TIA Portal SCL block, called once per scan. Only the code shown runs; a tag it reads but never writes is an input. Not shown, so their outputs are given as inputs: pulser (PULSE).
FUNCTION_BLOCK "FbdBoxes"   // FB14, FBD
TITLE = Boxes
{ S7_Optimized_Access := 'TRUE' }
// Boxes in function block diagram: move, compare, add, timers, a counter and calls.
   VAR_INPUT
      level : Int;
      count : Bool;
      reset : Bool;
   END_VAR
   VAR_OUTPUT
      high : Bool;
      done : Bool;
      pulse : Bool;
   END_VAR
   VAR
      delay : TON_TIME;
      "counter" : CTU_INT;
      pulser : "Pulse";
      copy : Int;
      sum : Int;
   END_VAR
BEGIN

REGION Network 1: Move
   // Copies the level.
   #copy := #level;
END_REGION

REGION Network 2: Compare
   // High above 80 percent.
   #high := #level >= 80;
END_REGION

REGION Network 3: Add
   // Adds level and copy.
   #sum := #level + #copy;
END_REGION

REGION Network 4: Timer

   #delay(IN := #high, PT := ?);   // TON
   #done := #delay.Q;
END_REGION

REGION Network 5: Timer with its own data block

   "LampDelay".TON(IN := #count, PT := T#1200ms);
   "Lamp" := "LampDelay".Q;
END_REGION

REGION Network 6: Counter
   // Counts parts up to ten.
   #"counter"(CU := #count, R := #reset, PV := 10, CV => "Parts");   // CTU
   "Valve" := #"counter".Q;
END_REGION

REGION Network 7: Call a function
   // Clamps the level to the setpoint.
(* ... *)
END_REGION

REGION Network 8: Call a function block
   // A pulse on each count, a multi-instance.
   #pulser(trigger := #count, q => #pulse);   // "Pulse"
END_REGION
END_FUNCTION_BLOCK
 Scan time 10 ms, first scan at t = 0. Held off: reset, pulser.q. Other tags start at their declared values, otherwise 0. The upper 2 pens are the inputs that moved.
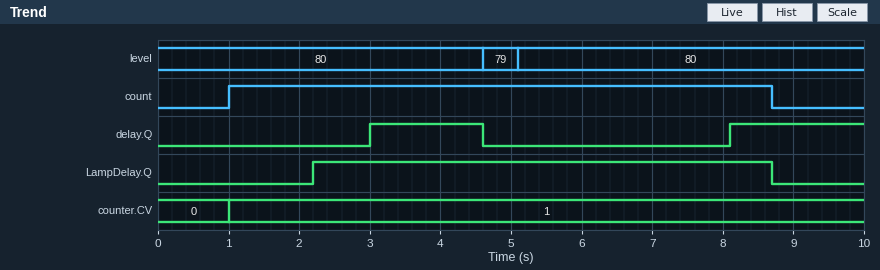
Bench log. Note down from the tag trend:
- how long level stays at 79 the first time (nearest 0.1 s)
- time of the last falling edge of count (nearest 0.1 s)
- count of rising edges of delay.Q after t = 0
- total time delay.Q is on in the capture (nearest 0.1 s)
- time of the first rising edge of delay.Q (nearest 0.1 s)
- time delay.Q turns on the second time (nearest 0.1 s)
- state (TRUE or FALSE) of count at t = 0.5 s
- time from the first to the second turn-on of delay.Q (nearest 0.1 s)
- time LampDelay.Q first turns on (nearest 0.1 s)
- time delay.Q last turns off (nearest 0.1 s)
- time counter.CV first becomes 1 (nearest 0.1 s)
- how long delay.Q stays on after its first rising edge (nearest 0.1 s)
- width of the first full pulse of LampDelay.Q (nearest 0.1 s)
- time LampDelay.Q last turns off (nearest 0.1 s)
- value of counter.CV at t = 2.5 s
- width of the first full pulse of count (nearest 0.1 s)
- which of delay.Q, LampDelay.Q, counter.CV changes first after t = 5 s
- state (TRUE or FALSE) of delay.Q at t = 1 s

0.5 s
8.7 s
2
3.5 s
3.0 s
8.1 s
FALSE
5.1 s
2.2 s
4.6 s
1.0 s
1.6 s
6.5 s
8.7 s
1
7.7 s
delay.Q
FALSE
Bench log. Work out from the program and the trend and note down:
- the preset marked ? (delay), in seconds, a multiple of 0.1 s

3.0 s
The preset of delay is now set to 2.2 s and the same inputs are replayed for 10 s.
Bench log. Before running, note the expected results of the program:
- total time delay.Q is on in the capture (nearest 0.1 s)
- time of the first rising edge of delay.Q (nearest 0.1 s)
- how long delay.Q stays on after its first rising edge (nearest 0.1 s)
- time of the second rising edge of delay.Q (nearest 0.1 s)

5.1 s
2.2 s
2.4 s
7.3 s
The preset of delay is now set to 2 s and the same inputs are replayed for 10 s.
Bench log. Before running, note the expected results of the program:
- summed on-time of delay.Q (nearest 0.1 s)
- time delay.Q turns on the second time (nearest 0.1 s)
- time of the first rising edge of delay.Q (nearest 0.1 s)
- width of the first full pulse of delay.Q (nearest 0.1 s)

5.5 s
7.1 s
2.0 s
2.6 s
